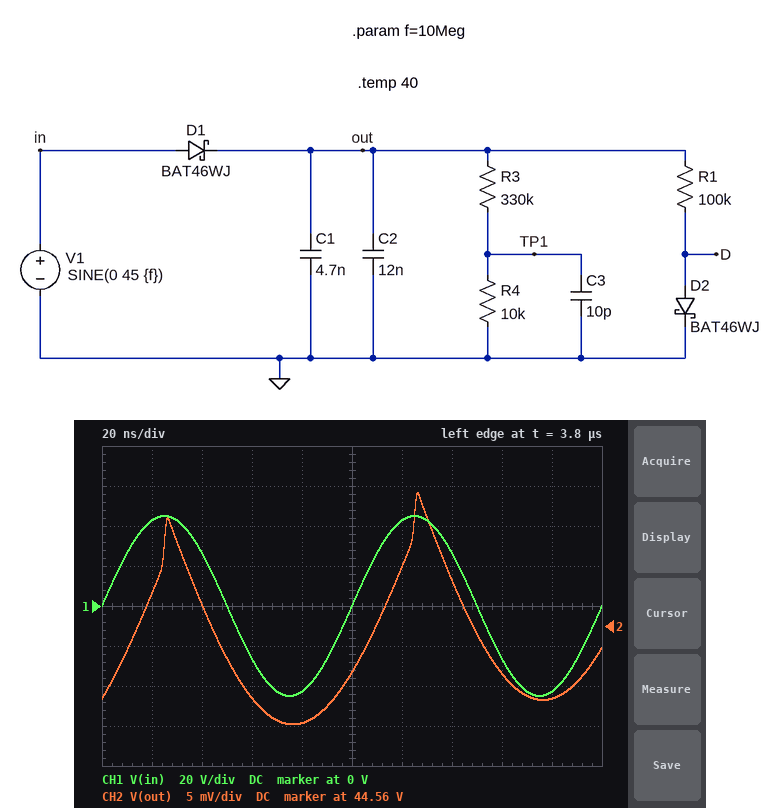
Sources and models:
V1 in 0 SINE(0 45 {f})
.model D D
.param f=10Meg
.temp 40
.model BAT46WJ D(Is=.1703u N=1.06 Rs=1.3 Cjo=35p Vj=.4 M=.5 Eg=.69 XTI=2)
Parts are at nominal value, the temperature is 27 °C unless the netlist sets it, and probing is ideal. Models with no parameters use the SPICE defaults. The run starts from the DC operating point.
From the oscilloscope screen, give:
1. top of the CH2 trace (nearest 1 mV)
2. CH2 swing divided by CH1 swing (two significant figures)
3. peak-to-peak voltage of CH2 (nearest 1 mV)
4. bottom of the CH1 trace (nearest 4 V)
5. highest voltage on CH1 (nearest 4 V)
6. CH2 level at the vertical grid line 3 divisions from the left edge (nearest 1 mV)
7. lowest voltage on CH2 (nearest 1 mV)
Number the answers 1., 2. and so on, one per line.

1. 44.582 V
2. 0.00032
3. 29 mV
4. -44 V
5. 44 V
6. 44.556 V
7. 44.553 V
